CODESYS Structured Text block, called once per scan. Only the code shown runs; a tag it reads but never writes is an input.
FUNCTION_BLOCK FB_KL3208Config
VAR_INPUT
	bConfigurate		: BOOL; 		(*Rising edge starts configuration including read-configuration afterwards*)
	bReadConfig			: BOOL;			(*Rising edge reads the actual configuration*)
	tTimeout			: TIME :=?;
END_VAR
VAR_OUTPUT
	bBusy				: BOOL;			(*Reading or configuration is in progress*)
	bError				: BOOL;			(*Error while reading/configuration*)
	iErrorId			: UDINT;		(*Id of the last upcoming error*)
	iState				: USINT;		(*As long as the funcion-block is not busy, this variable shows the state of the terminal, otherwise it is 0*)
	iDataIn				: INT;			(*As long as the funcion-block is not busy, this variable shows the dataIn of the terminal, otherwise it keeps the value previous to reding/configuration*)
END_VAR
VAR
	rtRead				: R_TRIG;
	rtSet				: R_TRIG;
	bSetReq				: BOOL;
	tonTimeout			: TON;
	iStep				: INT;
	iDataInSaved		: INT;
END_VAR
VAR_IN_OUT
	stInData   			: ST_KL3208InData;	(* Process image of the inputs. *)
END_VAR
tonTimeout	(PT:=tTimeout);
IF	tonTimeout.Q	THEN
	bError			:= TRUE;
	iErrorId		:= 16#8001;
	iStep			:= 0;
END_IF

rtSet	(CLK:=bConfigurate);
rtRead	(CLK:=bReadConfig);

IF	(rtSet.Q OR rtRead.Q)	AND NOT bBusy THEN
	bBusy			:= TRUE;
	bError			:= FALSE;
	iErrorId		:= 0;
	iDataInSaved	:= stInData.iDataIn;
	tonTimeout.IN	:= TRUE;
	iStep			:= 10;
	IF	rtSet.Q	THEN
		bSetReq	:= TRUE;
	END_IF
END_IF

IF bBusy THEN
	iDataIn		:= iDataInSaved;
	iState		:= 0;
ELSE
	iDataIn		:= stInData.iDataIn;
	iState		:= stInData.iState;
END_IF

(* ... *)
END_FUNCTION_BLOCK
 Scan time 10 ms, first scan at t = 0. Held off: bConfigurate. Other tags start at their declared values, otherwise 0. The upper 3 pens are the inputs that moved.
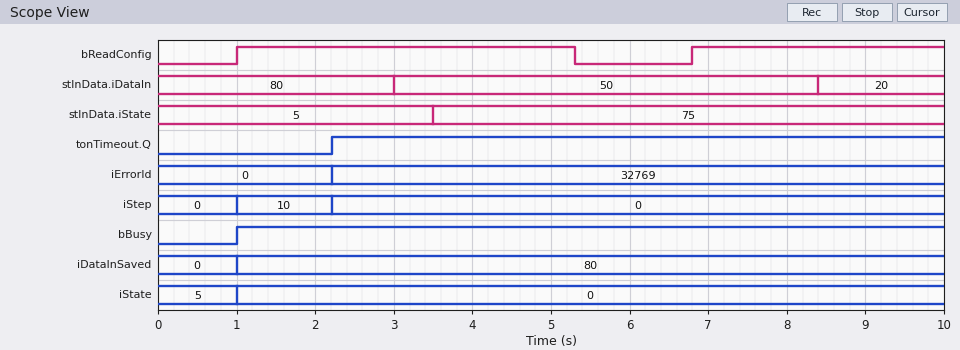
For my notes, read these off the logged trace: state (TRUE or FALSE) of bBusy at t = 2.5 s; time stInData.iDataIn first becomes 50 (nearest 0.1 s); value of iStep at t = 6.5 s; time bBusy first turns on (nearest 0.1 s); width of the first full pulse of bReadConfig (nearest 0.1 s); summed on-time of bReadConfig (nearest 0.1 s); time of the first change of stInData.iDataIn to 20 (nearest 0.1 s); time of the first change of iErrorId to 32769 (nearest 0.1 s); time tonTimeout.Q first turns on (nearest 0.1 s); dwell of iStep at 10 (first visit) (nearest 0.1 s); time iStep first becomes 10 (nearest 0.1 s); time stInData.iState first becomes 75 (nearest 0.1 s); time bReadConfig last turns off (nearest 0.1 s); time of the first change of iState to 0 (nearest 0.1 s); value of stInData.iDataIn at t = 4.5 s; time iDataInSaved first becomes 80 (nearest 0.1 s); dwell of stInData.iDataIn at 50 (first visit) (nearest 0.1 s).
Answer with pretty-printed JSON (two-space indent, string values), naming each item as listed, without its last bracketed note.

{
  "state (TRUE or FALSE) of bBusy at t = 2.5 s": "TRUE",
  "time stInData.iDataIn first becomes 50": "3.0 s",
  "value of iStep at t = 6.5 s": "0",
  "time bBusy first turns on": "1.0 s",
  "width of the first full pulse of bReadConfig": "4.3 s",
  "summed on-time of bReadConfig": "7.5 s",
  "time of the first change of stInData.iDataIn to 20": "8.4 s",
  "time of the first change of iErrorId to 32769": "2.2 s",
  "time tonTimeout.Q first turns on": "2.2 s",
  "dwell of iStep at 10 (first visit)": "1.2 s",
  "time iStep first becomes 10": "1.0 s",
  "time stInData.iState first becomes 75": "3.5 s",
  "time bReadConfig last turns off": "5.3 s",
  "time of the first change of iState to 0": "1.0 s",
  "value of stInData.iDataIn at t = 4.5 s": "50",
  "time iDataInSaved first becomes 80": "1.0 s",
  "dwell of stInData.iDataIn at 50 (first visit)": "5.4 s"
}
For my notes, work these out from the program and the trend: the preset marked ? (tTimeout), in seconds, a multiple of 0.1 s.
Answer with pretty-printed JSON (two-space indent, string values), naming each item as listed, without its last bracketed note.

{
  "the preset marked ? (tTimeout), in seconds, a multiple of 0.1 s": "1.2 s"
}
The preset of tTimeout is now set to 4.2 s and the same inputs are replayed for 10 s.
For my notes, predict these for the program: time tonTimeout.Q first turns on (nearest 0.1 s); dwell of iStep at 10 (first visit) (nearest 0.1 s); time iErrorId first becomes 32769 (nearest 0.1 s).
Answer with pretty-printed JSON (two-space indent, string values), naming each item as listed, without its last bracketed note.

{
  "time tonTimeout.Q first turns on": "5.2 s",
  "dwell of iStep at 10 (first visit)": "4.2 s",
  "time iErrorId first becomes 32769": "5.2 s"
}
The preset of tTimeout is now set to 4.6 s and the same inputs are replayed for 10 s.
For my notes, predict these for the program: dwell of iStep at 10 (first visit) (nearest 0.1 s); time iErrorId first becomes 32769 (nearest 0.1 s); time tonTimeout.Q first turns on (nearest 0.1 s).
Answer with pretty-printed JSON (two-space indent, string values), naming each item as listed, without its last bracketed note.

{
  "dwell of iStep at 10 (first visit)": "4.6 s",
  "time iErrorId first becomes 32769": "5.6 s",
  "time tonTimeout.Q first turns on": "5.6 s"
}
